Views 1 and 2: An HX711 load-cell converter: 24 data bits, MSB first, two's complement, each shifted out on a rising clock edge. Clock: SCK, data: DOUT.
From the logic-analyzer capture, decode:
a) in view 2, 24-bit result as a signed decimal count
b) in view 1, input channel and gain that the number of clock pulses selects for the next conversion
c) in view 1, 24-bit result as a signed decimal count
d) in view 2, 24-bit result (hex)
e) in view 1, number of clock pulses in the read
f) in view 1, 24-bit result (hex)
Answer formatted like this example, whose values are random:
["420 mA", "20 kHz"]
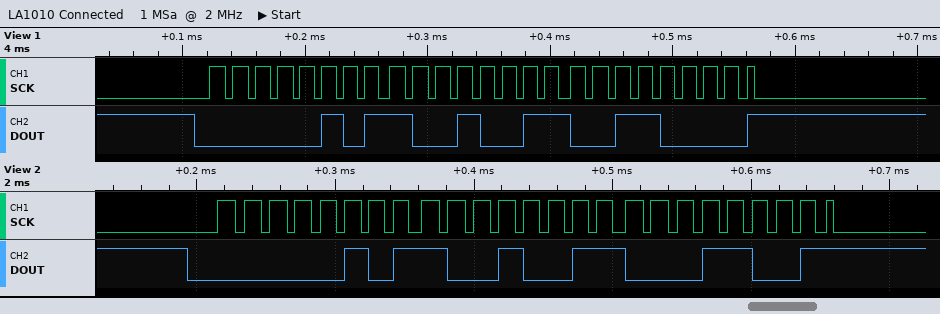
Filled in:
["365337", "channel A, gain 128", "365360", "0x059319", "25", "0x059330"]
